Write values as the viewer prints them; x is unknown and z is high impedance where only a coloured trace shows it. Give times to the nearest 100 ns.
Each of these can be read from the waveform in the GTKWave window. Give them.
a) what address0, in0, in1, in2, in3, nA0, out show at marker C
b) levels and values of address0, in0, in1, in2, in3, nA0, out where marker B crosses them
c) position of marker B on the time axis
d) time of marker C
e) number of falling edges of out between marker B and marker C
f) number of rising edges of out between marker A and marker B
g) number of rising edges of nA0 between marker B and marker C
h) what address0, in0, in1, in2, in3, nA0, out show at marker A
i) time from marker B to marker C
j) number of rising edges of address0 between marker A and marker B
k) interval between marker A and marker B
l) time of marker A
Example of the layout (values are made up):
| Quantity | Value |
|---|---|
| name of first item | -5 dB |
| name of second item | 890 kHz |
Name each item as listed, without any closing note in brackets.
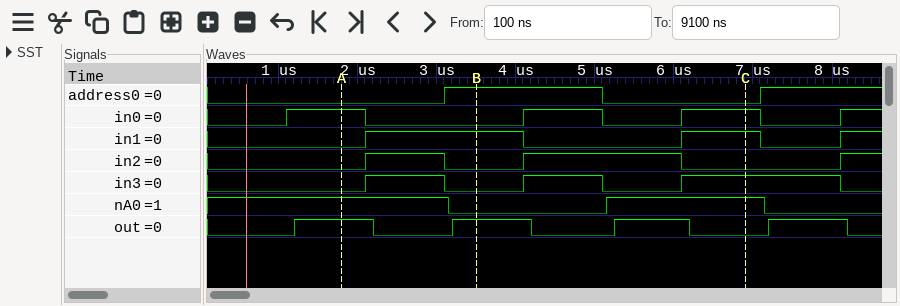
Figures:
| Quantity | Value |
|---|---|
| what address0, in0, in1, in2, in3, nA0, out show at marker C | address0=0, in0=1, in1=1, in2=0, in3=1, nA0=1, out=0 |
| levels and values of address0, in0, in1, in2, in3, nA0, out where marker B crosses them | address0=1, in0=0, in1=1, in2=0, in3=0, nA0=0, out=1 |
| position of marker B on the time axis | 3500 ns |
| time of marker C | 6900 ns |
| number of falling edges of out between marker B and marker C | 2 |
| number of rising edges of out between marker A and marker B | 1 |
| number of rising edges of nA0 between marker B and marker C | 1 |
| what address0, in0, in1, in2, in3, nA0, out show at marker A | address0=0, in0=1, in1=0, in2=0, in3=0, nA0=1, out=1 |
| time from marker B to marker C | 3400 ns |
| number of rising edges of address0 between marker A and marker B | 1 |
| interval between marker A and marker B | 1700 ns |
| time of marker A | 1800 ns |
